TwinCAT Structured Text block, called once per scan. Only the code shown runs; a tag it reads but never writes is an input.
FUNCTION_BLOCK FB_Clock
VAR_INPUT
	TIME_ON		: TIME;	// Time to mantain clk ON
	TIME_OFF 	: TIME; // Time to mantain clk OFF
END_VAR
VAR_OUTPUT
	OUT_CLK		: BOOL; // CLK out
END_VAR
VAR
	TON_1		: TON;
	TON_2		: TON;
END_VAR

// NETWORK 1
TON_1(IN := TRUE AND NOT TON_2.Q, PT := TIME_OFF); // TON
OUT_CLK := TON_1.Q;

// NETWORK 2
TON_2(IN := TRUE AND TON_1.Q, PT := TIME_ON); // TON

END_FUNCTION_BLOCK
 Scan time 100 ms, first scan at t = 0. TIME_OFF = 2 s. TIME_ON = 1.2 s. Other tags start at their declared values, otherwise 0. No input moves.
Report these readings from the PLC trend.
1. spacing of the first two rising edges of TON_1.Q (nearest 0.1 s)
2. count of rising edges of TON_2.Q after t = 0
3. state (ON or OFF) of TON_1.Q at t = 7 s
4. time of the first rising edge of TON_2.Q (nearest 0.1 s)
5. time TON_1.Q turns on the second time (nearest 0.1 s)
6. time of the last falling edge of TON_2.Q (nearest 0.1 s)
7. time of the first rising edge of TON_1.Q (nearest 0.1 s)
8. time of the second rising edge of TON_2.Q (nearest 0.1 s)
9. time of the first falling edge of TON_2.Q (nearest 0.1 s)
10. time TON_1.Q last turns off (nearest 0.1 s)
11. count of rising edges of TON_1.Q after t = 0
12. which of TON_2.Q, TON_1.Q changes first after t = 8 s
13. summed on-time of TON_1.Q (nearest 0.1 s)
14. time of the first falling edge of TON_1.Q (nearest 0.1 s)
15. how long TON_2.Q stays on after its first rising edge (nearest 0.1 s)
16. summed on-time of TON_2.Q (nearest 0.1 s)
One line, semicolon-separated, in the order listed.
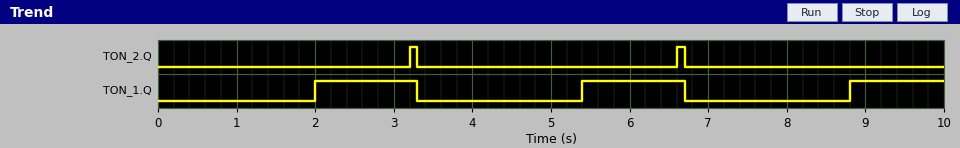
3.4 s; 2; OFF; 3.2 s; 5.4 s; 6.7 s; 2.0 s; 6.6 s; 3.3 s; 6.7 s; 3; TON_1.Q; 3.8 s; 3.3 s; 0.1 s; 0.2 s
